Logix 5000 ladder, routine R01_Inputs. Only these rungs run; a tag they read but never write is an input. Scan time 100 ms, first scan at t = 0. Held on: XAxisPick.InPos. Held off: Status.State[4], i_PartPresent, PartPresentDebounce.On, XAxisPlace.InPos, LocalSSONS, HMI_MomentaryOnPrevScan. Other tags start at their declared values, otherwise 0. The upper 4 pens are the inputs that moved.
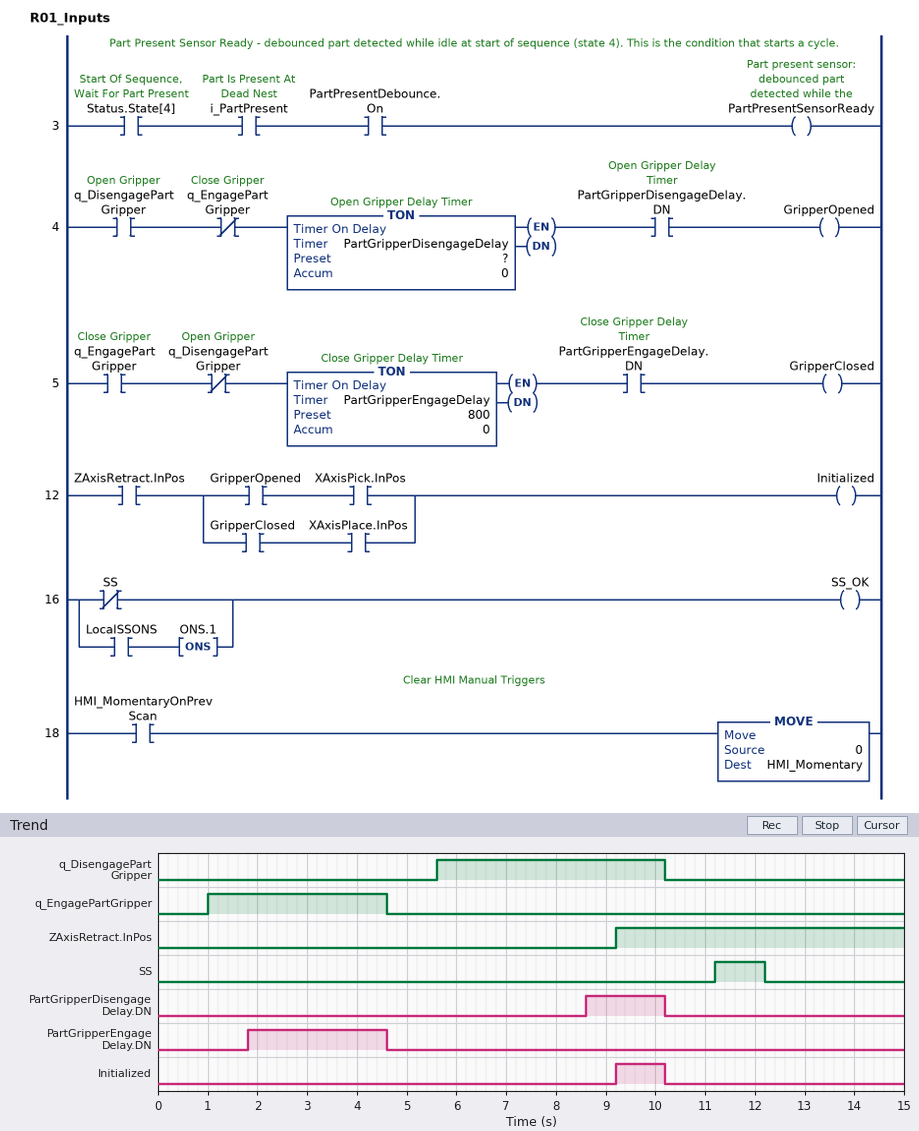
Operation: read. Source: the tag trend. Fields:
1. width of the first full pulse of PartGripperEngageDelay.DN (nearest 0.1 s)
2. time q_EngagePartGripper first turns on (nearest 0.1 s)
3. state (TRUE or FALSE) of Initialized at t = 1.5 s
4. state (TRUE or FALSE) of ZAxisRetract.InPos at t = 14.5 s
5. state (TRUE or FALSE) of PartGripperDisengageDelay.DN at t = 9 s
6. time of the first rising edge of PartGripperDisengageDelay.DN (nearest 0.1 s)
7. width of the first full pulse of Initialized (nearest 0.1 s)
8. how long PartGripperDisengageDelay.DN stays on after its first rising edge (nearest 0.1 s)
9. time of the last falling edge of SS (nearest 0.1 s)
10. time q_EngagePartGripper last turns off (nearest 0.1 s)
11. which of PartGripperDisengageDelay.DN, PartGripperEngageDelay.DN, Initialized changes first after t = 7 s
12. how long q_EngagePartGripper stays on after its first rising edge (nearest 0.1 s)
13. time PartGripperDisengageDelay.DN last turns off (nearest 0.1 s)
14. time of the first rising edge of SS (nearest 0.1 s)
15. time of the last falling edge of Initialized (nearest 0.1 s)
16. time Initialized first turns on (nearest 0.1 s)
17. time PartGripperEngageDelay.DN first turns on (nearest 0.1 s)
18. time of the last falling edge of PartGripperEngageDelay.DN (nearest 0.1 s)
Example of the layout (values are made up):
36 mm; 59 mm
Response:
2.8 s; 1.0 s; FALSE; TRUE; TRUE; 8.6 s; 1.0 s; 1.6 s; 12.2 s; 4.6 s; PartGripperDisengageDelay.DN; 3.6 s; 10.2 s; 11.2 s; 10.2 s; 9.2 s; 1.8 s; 4.6 s
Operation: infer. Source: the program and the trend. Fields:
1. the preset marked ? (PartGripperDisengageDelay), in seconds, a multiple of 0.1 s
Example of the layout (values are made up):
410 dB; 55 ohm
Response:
3.0 s
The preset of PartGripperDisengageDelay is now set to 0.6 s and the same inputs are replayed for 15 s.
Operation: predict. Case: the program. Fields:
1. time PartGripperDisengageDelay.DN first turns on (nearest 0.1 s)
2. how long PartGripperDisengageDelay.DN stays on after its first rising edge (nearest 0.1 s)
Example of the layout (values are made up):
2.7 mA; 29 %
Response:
6.2 s; 4.0 s
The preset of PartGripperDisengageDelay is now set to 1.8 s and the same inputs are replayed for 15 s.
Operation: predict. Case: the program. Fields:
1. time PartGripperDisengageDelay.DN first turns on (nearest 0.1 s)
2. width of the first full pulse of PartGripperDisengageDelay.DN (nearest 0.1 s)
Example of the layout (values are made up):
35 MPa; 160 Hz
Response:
7.4 s; 2.8 s
